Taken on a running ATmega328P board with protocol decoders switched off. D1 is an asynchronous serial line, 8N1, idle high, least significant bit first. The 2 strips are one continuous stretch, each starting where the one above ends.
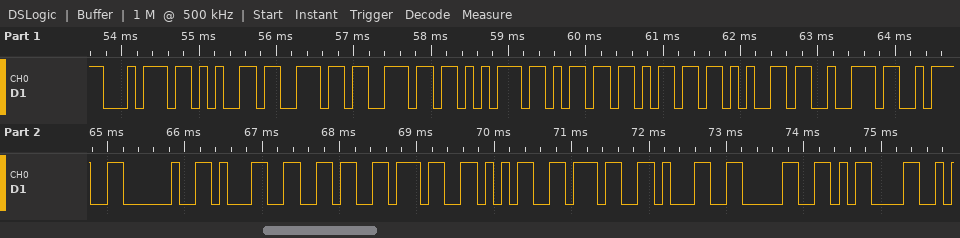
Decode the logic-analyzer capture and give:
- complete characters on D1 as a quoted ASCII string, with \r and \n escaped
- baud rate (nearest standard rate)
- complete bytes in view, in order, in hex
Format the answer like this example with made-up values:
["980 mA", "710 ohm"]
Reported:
["\"tennummer: 1675710\\r\"", "9600 baud", "74 65 6E 6E 75 6D 6D 65 72 3A 20 31 36 37 35 37 31 30 0D"]
